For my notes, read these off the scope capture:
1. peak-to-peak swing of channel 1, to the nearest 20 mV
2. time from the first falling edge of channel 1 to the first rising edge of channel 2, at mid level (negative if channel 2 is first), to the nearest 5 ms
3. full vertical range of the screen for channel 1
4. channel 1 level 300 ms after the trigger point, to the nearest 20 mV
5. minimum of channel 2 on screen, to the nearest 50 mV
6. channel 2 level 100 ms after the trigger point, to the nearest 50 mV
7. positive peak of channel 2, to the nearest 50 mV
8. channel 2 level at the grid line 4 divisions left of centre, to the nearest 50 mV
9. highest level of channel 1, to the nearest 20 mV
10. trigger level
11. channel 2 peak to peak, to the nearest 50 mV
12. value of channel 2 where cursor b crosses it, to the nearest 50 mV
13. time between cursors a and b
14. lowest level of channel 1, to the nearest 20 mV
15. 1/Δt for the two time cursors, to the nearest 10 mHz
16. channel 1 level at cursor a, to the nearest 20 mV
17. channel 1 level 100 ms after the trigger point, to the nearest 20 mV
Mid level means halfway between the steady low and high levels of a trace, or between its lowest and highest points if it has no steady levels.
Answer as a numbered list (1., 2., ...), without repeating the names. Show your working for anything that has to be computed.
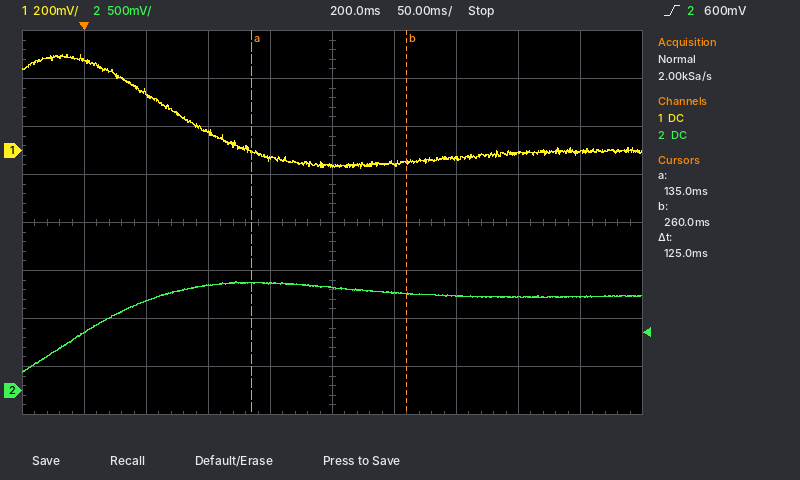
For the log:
1. 400 mV − (-80 mV) = 480 mV
2. -65 ms
3. 1.6 V
4. -40 mV
5. 200 mV
6. 1.10 V
7. 1.15 V
8. 600 mV
9. 400 mV
10. 600 mV
11. 1.15 V − (200 mV) = 950 mV
12. 1.00 V
13. 125 ms
14. -80 mV
15. 1 / 125 ms ≈ 8.00 Hz
16. 0 mV
17. 80 mV
